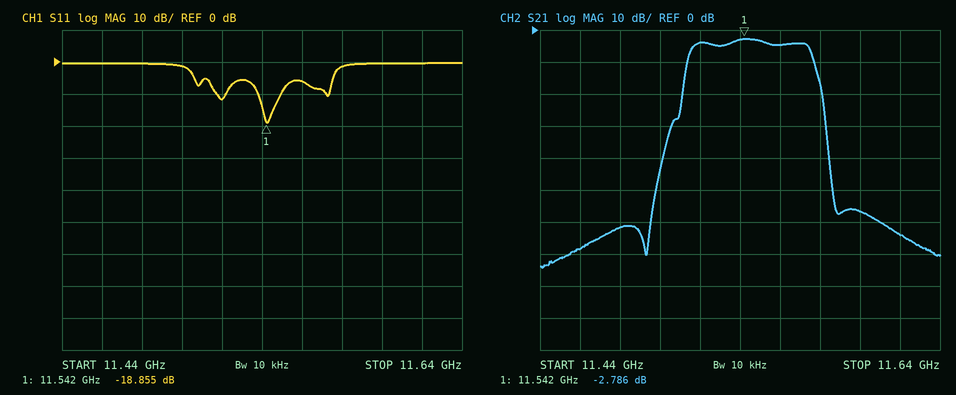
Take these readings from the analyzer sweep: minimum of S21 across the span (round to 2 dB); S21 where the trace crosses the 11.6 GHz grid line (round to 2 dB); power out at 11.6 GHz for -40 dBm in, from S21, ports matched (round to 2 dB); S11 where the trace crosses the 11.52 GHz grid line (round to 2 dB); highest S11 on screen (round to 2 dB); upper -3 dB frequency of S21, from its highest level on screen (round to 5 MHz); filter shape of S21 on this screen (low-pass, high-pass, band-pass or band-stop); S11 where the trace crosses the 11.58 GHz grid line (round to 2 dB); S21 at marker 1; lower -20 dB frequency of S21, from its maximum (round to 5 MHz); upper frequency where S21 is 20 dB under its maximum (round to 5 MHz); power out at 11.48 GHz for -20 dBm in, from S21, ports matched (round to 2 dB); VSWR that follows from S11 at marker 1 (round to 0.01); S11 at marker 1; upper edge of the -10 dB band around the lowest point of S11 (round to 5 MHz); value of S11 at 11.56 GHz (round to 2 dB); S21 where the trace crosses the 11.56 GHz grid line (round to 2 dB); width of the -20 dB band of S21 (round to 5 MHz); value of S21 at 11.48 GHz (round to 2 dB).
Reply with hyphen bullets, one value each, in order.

- -74 dB
- -56 dB
- -96 dBm
- -12 dB
- 0 dB
- 11.575 GHz
- band-pass
- -2 dB
- -2.786 dB
- 11.510 GHz
- 11.580 GHz
- -82 dBm
- 1.26
- -18.855 dB
- 11.550 GHz
- -6 dB
- -4 dB
- 70 MHz
- -62 dB
